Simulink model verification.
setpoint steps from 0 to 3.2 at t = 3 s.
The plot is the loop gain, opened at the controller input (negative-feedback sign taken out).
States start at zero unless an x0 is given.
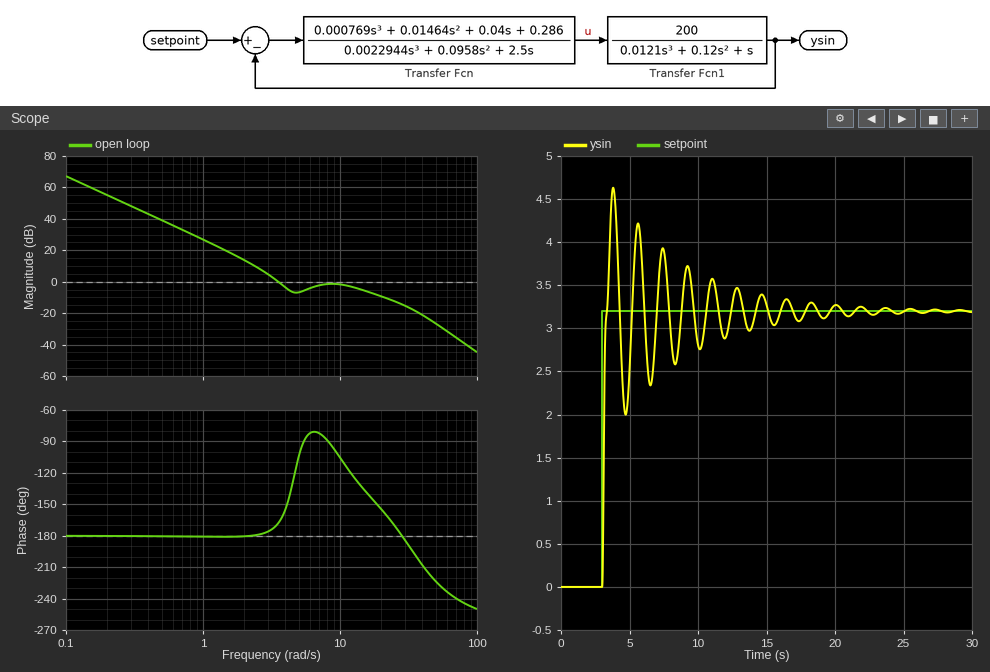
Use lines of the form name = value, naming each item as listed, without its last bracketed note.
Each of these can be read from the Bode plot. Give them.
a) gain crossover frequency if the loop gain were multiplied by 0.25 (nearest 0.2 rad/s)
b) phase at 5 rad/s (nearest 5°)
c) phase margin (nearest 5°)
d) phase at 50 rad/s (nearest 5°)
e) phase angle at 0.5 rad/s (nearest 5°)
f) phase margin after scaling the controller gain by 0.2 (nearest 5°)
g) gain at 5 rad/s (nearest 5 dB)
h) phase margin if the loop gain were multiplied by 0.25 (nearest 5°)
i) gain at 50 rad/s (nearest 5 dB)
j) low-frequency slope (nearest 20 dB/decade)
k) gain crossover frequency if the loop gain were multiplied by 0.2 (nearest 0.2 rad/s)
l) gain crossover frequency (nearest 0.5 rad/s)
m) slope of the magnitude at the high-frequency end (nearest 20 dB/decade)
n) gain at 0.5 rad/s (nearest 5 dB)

gain crossover frequency if the loop gain were multiplied by 0.25 = 2.2 rad/s
phase at 5 rad/s = -105°
phase margin = 10°
phase at 50 rad/s = -225°
phase angle at 0.5 rad/s = -180°
phase margin after scaling the controller gain by 0.2 = 0°
gain at 5 rad/s = -5 dB
phase margin if the loop gain were multiplied by 0.25 = 0°
gain at 50 rad/s = -25 dB
low-frequency slope = -40 dB/decade
gain crossover frequency if the loop gain were multiplied by 0.2 = 2.0 rad/s
gain crossover frequency = 3.5 rad/s
slope of the magnitude at the high-frequency end = -60 dB/decade
gain at 0.5 rad/s = 40 dB
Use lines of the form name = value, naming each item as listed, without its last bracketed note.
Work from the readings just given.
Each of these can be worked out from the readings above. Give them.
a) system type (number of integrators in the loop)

system type = 2
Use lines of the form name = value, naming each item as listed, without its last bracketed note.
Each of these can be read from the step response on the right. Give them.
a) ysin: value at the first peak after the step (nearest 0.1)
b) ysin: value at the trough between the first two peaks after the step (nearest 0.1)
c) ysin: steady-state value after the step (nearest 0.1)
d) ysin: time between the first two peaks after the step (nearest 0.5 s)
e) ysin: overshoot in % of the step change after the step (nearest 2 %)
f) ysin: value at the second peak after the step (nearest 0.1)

ysin: value at the first peak after the step = 4.6
ysin: value at the trough between the first two peaks after the step = 2.0
ysin: steady-state value after the step = 3.2
ysin: time between the first two peaks after the step = 2.0 s
ysin: overshoot in % of the step change after the step = 44 %
ysin: value at the second peak after the step = 4.2
